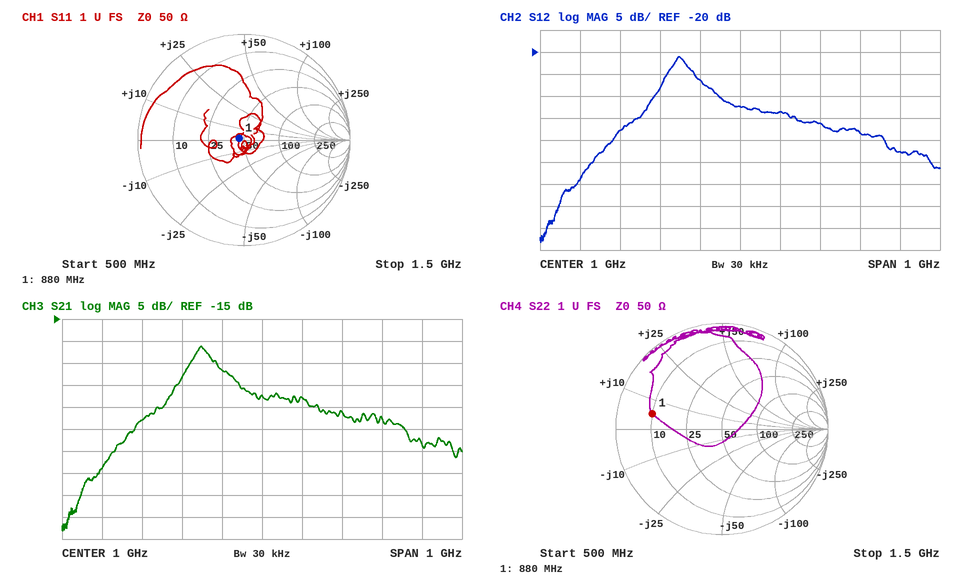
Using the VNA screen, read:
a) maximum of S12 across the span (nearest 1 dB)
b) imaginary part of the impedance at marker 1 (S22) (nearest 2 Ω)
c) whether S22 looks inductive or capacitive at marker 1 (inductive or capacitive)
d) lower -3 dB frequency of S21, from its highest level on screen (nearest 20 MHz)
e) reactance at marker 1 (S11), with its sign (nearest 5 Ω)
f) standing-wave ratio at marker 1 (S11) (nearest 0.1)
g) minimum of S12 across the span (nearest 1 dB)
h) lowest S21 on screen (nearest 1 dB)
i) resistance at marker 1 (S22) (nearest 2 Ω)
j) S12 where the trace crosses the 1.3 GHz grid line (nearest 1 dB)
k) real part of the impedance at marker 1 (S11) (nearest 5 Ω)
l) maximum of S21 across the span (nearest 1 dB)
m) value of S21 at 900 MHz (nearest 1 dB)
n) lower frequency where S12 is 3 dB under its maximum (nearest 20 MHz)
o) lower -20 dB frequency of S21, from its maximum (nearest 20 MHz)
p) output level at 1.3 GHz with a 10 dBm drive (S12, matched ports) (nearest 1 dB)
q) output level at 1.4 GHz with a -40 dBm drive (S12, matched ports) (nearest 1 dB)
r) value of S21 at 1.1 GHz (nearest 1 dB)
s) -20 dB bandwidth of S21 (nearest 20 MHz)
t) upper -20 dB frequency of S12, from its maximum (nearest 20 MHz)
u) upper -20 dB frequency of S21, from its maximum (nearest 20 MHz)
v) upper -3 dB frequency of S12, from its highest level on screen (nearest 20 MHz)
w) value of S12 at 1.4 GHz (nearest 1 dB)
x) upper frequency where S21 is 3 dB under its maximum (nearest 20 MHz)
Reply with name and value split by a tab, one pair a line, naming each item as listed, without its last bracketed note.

maximum of S12 across the span	-21 dB
imaginary part of the impedance at marker 1 (S22)	+6 Ω
whether S22 looks inductive or capacitive at marker 1	inductive
lower -3 dB frequency of S21, from its highest level on screen	820 MHz
reactance at marker 1 (S11), with its sign	0 Ω
standing-wave ratio at marker 1 (S11)	1.1
minimum of S12 across the span	-63 dB
lowest S21 on screen	-63 dB
resistance at marker 1 (S22)	10 Ω
S12 where the trace crosses the 1.3 GHz grid line	-38 dB
real part of the impedance at marker 1 (S11)	45 Ω
maximum of S21 across the span	-21 dB
value of S21 at 900 MHz	-27 dB
lower frequency where S12 is 3 dB under its maximum	820 MHz
lower -20 dB frequency of S21, from its maximum	660 MHz
output level at 1.3 GHz with a 10 dBm drive (S12, matched ports)	-28 dBm
output level at 1.4 GHz with a -40 dBm drive (S12, matched ports)	-83 dBm
value of S21 at 1.1 GHz	-33 dB
-20 dB bandwidth of S21	700 MHz
upper -20 dB frequency of S12, from its maximum	1.36 GHz
upper -20 dB frequency of S21, from its maximum	1.36 GHz
upper -3 dB frequency of S12, from its highest level on screen	880 MHz
value of S12 at 1.4 GHz	-43 dB
upper frequency where S21 is 3 dB under its maximum	880 MHz
